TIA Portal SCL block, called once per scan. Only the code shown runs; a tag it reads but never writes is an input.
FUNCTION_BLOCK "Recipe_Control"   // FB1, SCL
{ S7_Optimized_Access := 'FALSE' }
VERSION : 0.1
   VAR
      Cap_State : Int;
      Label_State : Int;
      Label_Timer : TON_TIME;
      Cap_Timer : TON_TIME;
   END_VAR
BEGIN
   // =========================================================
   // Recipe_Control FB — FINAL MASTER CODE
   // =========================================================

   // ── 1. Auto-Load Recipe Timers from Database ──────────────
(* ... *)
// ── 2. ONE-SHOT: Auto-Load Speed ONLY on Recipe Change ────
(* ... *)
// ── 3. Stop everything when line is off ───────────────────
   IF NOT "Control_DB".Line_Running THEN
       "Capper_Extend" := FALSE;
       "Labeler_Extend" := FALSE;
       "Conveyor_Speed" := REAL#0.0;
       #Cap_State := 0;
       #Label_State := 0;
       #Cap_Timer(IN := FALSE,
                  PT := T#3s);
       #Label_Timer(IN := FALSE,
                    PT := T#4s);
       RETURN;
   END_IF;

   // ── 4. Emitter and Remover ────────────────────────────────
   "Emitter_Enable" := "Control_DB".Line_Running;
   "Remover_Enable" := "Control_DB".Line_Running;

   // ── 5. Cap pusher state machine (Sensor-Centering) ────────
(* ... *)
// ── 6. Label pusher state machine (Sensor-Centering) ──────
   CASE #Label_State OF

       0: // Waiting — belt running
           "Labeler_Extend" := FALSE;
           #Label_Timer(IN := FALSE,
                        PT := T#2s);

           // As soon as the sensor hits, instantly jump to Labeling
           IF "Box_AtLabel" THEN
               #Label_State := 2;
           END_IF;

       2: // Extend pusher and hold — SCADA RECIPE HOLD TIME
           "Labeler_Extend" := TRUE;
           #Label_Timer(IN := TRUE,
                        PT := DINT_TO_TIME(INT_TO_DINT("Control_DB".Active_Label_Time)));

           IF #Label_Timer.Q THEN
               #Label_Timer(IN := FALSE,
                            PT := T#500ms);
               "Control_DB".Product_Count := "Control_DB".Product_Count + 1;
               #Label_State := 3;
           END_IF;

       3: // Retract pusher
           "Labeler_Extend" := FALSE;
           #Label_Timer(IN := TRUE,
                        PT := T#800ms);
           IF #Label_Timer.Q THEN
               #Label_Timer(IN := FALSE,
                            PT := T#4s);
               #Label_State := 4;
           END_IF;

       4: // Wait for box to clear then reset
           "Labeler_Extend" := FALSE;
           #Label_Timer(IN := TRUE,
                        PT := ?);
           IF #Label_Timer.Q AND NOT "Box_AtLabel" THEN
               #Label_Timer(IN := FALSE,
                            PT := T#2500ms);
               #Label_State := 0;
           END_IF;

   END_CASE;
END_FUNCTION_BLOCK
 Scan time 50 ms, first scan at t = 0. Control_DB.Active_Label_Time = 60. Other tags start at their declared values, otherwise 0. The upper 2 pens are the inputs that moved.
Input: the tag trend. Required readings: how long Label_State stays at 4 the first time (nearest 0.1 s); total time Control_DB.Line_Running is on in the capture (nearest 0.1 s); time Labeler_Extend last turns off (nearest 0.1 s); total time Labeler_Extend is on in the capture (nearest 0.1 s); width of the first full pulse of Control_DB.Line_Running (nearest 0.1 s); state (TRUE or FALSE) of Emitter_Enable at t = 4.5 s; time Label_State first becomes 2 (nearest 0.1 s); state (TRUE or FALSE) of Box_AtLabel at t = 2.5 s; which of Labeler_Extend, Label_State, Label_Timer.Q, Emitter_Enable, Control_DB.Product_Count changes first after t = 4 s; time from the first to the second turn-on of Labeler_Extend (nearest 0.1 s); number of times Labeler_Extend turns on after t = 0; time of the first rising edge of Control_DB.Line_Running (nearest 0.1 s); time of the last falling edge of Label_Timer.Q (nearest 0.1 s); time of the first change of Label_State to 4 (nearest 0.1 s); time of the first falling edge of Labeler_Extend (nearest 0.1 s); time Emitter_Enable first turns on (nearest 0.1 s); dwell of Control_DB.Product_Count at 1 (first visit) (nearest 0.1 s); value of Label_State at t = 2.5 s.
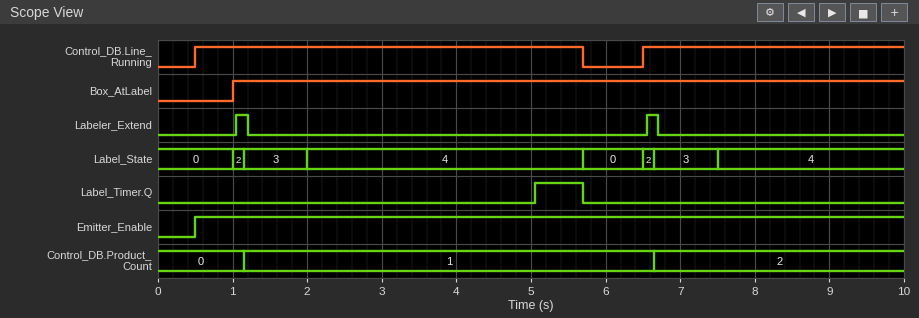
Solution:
3.7 s
8.7 s
6.7 s
0.3 s
5.2 s
TRUE
1.0 s
TRUE
Label_Timer.Q
5.5 s
2
0.5 s
5.7 s
2.0 s
1.2 s
0.5 s
5.5 s
4
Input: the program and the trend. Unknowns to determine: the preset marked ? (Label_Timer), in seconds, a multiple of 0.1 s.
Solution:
3.0 s
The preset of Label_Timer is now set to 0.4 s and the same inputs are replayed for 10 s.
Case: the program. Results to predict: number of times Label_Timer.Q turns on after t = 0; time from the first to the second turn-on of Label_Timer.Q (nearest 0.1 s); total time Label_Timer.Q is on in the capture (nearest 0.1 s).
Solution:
2
5.5 s
5.3 s
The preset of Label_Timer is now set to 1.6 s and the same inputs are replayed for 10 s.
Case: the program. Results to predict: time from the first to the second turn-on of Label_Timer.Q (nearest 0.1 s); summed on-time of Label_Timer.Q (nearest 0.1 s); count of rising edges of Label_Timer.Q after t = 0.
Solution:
5.5 s
2.9 s
2
